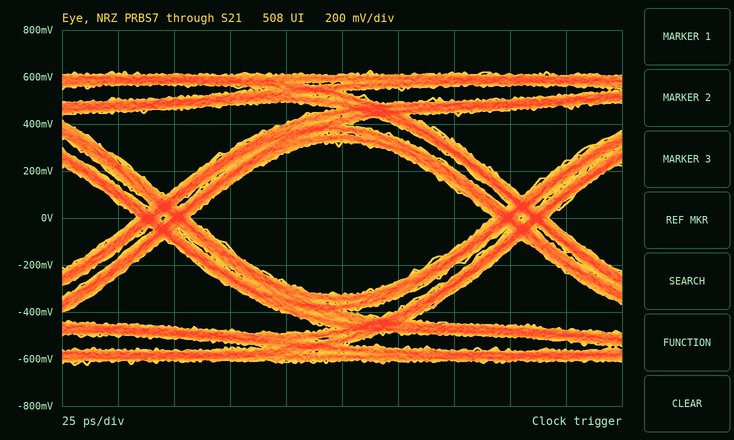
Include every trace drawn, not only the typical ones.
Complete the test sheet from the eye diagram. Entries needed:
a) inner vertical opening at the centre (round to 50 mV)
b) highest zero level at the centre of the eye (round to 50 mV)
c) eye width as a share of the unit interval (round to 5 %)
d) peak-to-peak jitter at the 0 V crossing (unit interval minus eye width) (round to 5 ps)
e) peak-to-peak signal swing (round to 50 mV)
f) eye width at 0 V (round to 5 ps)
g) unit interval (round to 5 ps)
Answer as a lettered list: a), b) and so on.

a) 650 mV
b) -350 mV
c) 85 %
d) 25 ps
e) 1.25 V
f) 135 ps
g) 160 ps
